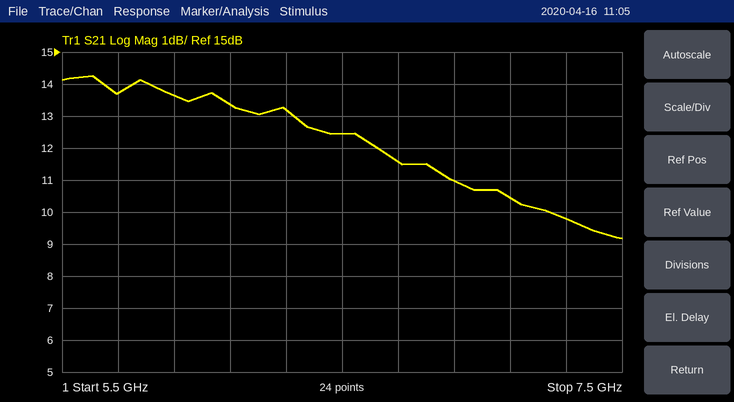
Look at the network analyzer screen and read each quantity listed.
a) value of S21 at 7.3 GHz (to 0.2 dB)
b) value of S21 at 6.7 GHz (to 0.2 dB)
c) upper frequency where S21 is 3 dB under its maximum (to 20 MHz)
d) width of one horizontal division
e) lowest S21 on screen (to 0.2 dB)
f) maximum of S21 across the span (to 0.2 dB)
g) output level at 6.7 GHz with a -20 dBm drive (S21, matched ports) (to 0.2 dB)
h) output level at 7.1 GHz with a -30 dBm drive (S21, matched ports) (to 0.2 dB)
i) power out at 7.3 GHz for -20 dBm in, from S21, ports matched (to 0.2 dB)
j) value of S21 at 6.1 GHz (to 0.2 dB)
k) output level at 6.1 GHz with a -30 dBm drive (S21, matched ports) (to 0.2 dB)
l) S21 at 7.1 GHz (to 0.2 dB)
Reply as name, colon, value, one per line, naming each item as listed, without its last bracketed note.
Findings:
value of S21 at 7.3 GHz: 9.8 dB
value of S21 at 6.7 GHz: 11.6 dB
upper frequency where S21 is 3 dB under its maximum: 6.84 GHz
width of one horizontal division: 200 MHz
lowest S21 on screen: 9.2 dB
maximum of S21 across the span: 14.2 dB
output level at 6.7 GHz with a -20 dBm drive (S21, matched ports): -8.4 dBm
output level at 7.1 GHz with a -30 dBm drive (S21, matched ports): -19.6 dBm
power out at 7.3 GHz for -20 dBm in, from S21, ports matched: -10.2 dBm
value of S21 at 6.1 GHz: 13.4 dB
output level at 6.1 GHz with a -30 dBm drive (S21, matched ports): -16.6 dBm
S21 at 7.1 GHz: 10.4 dB
